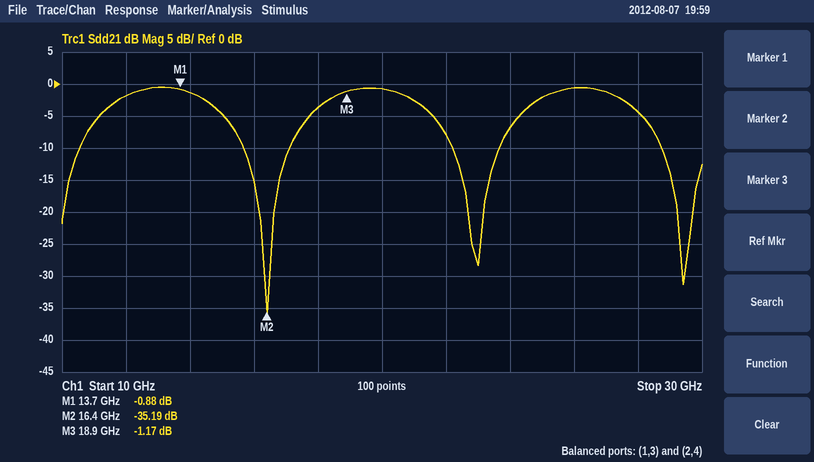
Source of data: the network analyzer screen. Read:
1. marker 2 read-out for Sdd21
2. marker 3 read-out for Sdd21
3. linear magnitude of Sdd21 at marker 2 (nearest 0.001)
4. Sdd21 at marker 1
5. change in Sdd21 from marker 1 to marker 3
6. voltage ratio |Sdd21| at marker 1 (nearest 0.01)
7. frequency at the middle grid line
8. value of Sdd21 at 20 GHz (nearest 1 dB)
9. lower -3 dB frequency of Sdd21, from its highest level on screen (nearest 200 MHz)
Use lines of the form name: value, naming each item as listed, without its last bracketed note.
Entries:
marker 2 read-out for Sdd21: -35.19 dB
marker 3 read-out for Sdd21: -1.17 dB
linear magnitude of Sdd21 at marker 2: 0.017
Sdd21 at marker 1: -0.88 dB
change in Sdd21 from marker 1 to marker 3: -0.29 dB
voltage ratio |Sdd21| at marker 1: 0.90
frequency at the middle grid line: 20 GHz
value of Sdd21 at 20 GHz: -1 dB
lower -3 dB frequency of Sdd21, from its highest level on screen: 11.4 GHz
